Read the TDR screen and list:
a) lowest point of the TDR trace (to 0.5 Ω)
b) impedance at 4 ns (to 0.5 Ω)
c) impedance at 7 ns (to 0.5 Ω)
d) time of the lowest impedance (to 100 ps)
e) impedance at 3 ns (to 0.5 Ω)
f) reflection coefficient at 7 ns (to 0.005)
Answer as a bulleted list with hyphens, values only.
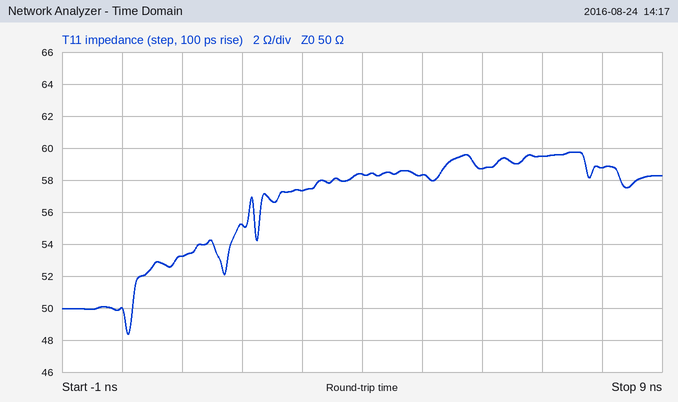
- 48.5 Ω
- 58.5 Ω
- 59.5 Ω
- 100 ps
- 57.5 Ω
- +0.085
